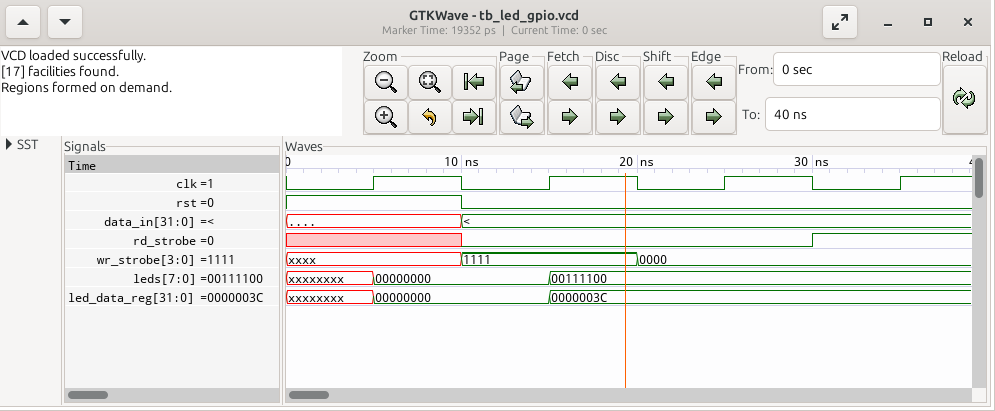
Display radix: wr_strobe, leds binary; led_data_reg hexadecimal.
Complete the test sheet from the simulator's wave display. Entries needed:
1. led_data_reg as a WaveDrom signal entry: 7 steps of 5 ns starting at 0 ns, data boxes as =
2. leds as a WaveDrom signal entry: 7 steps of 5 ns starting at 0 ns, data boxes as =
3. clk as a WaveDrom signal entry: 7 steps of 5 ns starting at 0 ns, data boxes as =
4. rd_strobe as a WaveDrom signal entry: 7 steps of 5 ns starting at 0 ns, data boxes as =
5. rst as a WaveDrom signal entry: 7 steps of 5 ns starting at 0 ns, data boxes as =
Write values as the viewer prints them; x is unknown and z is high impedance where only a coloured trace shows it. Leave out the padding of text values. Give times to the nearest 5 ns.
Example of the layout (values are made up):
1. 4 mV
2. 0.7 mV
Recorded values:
1. {name: 'led_data_reg', wave: 'x=.=...', data: '00000000 0000003C'}
2. {name: 'leds', wave: 'x=.=...', data: '00000000 00111100'}
3. {name: 'clk', wave: '0101010'}
4. {name: 'rd_strobe', wave: 'x.0...1'}
5. {name: 'rst', wave: '1.0....'}
